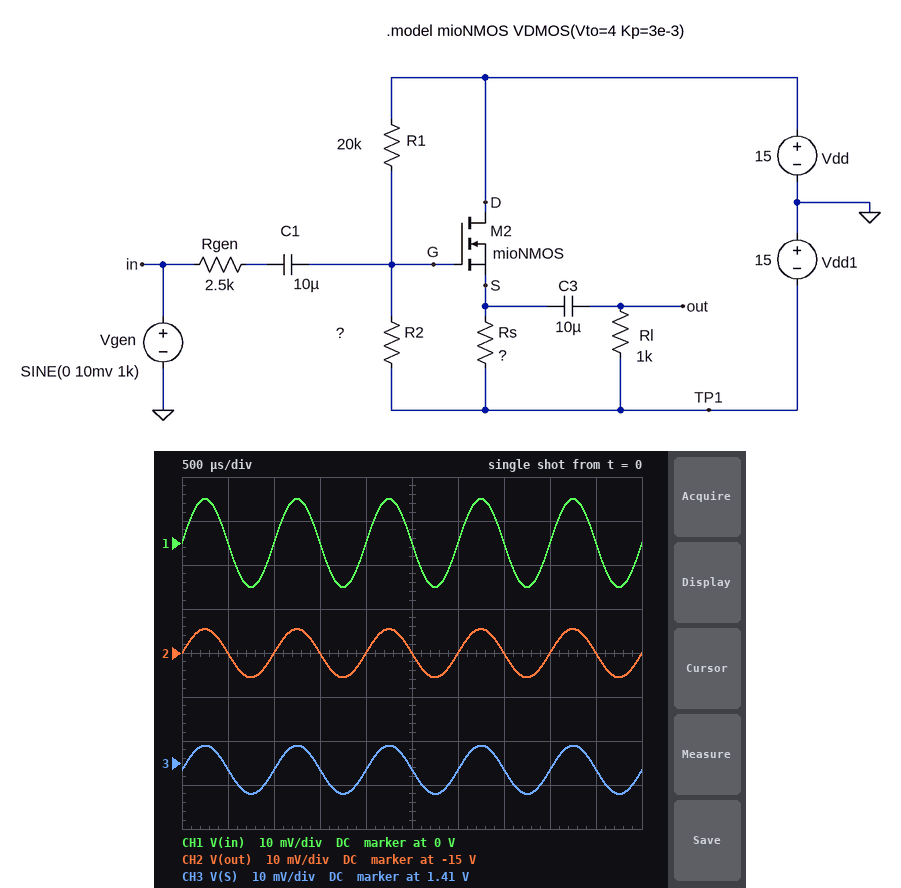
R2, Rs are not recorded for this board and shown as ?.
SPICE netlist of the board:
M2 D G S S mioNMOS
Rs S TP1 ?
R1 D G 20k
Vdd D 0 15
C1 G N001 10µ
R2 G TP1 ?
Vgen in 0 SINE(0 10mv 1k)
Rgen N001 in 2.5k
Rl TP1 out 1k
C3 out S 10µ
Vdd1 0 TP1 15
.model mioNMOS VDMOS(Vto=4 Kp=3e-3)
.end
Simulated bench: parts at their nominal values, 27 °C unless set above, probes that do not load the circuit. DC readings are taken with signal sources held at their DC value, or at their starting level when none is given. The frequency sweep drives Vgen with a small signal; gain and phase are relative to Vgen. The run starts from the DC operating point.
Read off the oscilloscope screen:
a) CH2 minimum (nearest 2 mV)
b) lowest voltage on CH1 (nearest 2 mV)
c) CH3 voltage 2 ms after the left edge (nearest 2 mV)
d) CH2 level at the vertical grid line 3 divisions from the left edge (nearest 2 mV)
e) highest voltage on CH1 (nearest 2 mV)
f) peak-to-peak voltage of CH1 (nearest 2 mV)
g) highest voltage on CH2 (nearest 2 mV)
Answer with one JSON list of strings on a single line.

["-15.006 V", "-10 mV", "1.408 V", "-15.000 V", "10 mV", "20 mV", "-14.994 V"]
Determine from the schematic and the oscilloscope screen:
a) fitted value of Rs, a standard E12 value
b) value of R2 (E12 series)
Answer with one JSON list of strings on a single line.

["27 kΩ", "47 kΩ"]
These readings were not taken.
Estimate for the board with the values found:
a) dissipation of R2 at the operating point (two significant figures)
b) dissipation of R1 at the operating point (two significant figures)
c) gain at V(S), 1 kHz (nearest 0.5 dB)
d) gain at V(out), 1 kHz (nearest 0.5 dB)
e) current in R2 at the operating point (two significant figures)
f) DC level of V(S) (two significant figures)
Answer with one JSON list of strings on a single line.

["9.4 mW", "4.0 mW", "-5.0 dB", "-5.0 dB", "450 µA", "1.4 V"]
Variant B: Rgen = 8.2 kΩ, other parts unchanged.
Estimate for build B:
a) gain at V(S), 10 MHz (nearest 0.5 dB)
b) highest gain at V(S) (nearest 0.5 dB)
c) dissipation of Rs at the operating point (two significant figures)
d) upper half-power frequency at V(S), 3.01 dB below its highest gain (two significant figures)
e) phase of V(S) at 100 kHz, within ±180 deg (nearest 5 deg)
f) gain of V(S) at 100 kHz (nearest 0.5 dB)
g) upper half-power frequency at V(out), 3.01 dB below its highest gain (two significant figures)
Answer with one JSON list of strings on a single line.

["-41.5 dB", "-4.5 dB", "10 mW", "59 Hz", "-45 deg", "-14.5 dB", "48 kHz"]
